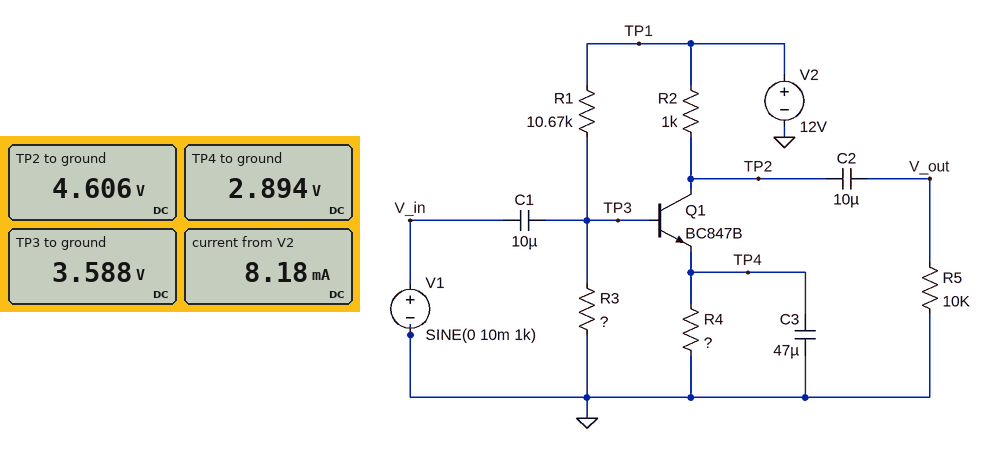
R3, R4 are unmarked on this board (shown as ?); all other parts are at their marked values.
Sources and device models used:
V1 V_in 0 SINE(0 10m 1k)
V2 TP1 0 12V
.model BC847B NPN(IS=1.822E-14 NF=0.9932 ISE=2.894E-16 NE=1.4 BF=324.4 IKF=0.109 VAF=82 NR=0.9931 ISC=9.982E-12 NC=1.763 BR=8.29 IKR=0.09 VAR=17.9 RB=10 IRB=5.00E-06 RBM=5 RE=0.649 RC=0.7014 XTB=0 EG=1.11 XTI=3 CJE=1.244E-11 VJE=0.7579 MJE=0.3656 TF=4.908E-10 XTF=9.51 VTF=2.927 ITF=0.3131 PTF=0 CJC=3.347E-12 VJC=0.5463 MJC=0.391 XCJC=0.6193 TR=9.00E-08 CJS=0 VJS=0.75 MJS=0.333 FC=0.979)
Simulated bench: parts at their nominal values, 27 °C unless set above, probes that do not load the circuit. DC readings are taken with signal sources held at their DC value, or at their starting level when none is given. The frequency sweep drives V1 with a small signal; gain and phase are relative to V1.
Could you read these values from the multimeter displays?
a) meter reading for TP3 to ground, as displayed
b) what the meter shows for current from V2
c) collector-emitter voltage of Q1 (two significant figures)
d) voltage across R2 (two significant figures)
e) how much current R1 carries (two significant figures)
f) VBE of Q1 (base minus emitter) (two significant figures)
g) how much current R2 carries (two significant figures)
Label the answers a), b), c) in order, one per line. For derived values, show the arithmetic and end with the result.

a) 3.588 V
b) 8.18 mA
c) 4.606 V - 2.894 V = 1.7 V
d) 12 V - 4.606 V = 7.4 V
e) (12 V - 3.588 V) / 10.67 kΩ = 790 µA
f) 3.588 V - 2.894 V = 690 mV
g) (12 V - 4.606 V) / 1 kΩ = 7.4 mA
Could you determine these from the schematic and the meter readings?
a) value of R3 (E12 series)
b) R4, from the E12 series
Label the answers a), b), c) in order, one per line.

a) 4.7 kΩ
b) 390 Ω
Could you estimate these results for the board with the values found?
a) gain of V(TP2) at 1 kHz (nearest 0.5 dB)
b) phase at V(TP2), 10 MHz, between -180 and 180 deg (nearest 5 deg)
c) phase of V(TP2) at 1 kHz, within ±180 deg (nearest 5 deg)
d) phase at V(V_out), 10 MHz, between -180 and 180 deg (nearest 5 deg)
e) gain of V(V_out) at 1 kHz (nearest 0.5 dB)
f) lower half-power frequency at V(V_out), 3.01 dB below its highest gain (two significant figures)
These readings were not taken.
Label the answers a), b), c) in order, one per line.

a) 44.0 dB
b) 165 deg
c) -145 deg
d) 165 deg
e) 44.0 dB
f) 750 Hz
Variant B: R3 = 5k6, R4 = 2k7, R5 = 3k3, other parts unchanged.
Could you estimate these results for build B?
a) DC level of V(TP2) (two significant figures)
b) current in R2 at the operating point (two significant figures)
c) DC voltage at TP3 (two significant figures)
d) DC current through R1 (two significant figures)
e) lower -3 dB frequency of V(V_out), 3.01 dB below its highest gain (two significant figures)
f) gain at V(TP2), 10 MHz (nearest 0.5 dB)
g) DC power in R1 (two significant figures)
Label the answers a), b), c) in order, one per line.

a) 11 V
b) 1.3 mA
c) 4.1 V
d) 740 µA
e) 160 Hz
f) 31.0 dB
g) 5.8 mW
